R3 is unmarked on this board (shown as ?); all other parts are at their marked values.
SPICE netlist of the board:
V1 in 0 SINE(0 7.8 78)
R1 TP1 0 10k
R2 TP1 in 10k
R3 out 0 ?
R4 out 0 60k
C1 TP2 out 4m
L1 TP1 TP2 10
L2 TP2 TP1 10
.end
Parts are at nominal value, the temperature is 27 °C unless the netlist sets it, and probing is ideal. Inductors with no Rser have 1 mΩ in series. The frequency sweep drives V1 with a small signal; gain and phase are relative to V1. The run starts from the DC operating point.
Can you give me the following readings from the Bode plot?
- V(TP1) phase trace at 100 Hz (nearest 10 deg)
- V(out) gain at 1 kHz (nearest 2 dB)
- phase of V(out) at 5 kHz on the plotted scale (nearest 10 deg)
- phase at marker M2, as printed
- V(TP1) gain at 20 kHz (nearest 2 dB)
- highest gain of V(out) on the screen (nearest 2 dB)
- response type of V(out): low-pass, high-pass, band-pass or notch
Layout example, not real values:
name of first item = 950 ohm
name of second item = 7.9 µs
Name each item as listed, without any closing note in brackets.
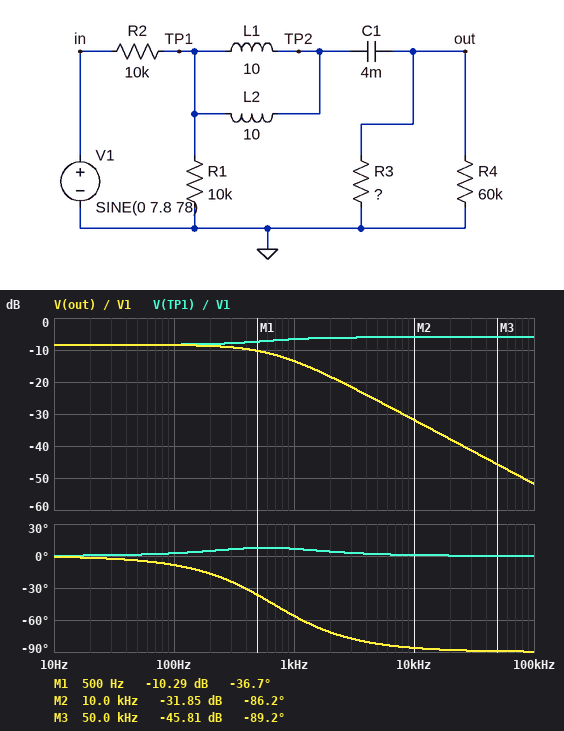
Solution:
V(TP1) phase trace at 100 Hz = 0 deg
V(out) gain at 1 kHz = -14 dB
phase of V(out) at 5 kHz on the plotted scale = -80 deg
phase at marker M2, as printed = -86.2 deg
V(TP1) gain at 20 kHz = -6 dB
highest gain of V(out) on the screen = -8 dB
response type of V(out): low-pass, high-pass, band-pass or notch = low-pass
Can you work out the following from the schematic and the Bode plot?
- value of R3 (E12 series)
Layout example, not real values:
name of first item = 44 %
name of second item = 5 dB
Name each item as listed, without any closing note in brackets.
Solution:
value of R3 = 22 kΩ
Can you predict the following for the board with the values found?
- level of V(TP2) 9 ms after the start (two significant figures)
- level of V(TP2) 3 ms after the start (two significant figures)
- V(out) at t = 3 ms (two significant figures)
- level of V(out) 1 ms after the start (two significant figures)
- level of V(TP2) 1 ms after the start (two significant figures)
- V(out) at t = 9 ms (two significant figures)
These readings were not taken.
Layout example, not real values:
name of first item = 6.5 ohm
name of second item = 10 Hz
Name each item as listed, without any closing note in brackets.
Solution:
level of V(TP2) 9 ms after the start = -2.7 V
level of V(TP2) 3 ms after the start = 2.9 V
V(out) at t = 3 ms = 2.9 V
level of V(out) 1 ms after the start = 1.1 V
level of V(TP2) 1 ms after the start = 1.1 V
V(out) at t = 9 ms = -2.7 V
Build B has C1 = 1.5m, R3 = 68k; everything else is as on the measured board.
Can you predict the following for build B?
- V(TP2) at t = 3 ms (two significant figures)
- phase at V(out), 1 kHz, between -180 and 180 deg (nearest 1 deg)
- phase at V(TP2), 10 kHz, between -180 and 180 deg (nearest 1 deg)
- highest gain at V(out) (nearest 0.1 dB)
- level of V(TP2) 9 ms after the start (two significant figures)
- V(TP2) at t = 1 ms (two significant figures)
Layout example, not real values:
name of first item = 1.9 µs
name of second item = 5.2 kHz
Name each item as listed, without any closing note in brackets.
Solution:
V(TP2) at t = 3 ms = 3.3 V
phase at V(out), 1 kHz, between -180 and 180 deg = -40 deg
phase at V(TP2), 10 kHz, between -180 and 180 deg = -83 deg
highest gain at V(out) = -7.3 dB
level of V(TP2) 9 ms after the start = -3.1 V
V(TP2) at t = 1 ms = 1.4 V
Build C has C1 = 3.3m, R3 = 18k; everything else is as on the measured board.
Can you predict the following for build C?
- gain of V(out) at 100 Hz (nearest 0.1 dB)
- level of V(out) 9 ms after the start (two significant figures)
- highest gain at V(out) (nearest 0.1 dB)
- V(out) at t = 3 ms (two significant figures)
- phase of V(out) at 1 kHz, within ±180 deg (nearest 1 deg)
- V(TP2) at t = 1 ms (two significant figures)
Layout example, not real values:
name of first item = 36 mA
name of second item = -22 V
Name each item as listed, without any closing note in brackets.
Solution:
gain of V(out) at 100 Hz = -8.8 dB
level of V(out) 9 ms after the start = -2.6 V
highest gain at V(out) = -8.7 dB
V(out) at t = 3 ms = 2.8 V
phase of V(out) at 1 kHz, within ±180 deg = -59 deg
V(TP2) at t = 1 ms = 1.0 V
